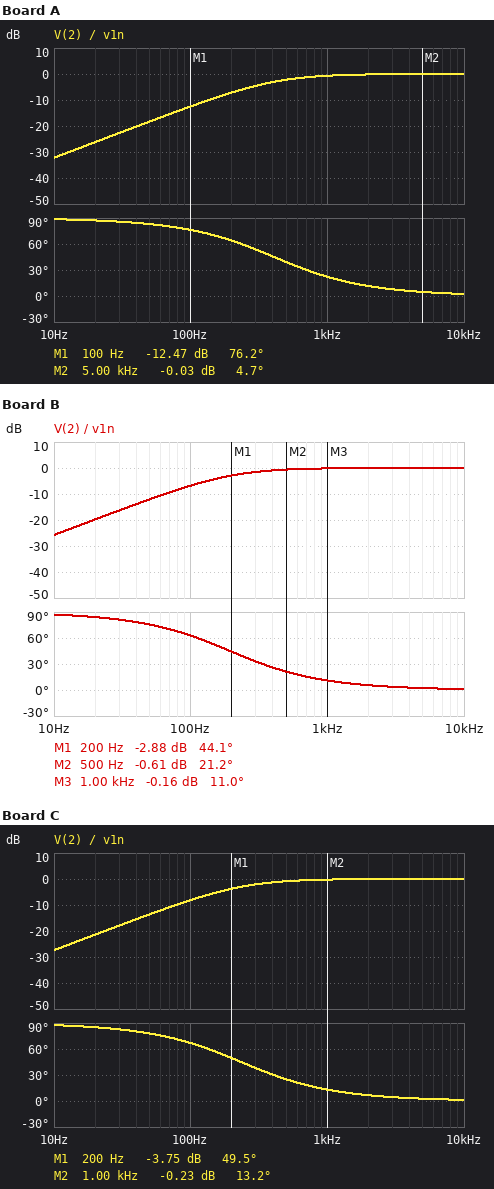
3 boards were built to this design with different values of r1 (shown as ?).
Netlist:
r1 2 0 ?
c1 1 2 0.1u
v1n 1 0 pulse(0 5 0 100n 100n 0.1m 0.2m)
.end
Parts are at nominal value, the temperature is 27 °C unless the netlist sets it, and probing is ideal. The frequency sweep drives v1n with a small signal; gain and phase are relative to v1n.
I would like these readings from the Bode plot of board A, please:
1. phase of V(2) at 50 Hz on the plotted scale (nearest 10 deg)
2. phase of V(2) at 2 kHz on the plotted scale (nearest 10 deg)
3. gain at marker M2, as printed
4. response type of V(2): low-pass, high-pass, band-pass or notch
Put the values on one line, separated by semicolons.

80 deg; 10 deg; -0.03 dB; high-pass
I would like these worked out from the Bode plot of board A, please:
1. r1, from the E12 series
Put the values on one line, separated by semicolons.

3.9 kΩ
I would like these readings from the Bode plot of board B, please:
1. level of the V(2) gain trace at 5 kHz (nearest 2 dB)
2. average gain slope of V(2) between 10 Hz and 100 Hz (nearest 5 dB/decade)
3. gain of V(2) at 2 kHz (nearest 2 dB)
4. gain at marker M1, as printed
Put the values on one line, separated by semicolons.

0 dB; 20 dB/decade; 0 dB; -2.88 dB
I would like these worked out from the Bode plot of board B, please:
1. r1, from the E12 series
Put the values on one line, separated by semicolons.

8.2 kΩ
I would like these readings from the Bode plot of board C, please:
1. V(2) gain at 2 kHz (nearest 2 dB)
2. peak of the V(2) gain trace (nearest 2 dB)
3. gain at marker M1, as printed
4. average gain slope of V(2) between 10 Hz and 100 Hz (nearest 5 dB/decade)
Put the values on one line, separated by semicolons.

0 dB; 0 dB; -3.75 dB; 20 dB/decade
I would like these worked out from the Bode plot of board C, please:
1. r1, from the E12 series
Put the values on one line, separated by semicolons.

6.8 kΩ
